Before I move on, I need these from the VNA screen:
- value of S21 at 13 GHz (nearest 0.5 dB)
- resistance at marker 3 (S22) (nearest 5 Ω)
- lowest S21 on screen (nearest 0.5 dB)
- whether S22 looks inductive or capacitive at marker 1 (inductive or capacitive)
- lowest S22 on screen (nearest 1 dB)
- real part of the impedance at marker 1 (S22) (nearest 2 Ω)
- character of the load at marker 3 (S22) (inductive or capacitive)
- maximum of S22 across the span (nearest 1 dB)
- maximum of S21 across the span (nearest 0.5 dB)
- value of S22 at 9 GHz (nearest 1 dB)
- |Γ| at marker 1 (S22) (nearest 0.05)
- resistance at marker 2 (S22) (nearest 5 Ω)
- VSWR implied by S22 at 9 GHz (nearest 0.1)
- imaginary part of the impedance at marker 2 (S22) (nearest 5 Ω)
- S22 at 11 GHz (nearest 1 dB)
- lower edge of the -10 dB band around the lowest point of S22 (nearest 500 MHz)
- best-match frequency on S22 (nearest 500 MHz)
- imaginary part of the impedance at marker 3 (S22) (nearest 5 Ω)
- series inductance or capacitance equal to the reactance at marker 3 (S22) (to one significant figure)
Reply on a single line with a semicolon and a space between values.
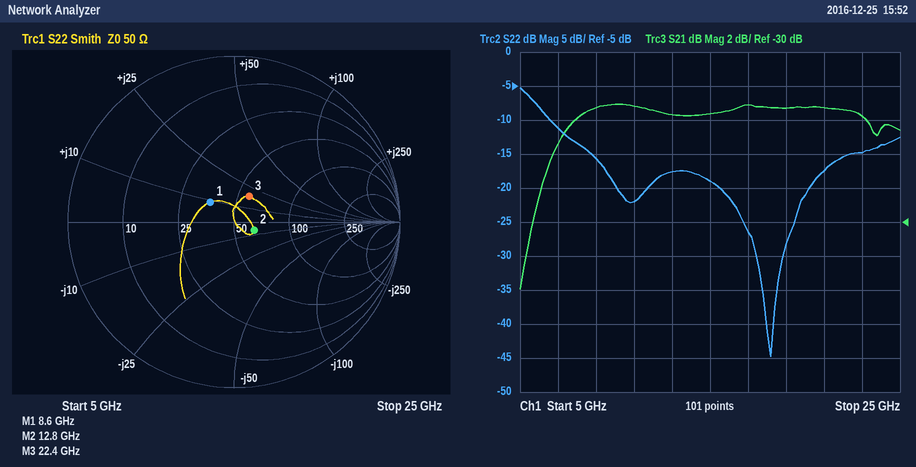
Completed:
-23.5 dB; 55 Ω; -34.0 dB; inductive; -45 dB; 36 Ω; inductive; -5 dB; -23.0 dB; -16 dB; 0.20; 65 Ω; 1.4; -5 Ω; -22 dB; 6.5 GHz; 18.0 GHz; +20 Ω; 100 pH
